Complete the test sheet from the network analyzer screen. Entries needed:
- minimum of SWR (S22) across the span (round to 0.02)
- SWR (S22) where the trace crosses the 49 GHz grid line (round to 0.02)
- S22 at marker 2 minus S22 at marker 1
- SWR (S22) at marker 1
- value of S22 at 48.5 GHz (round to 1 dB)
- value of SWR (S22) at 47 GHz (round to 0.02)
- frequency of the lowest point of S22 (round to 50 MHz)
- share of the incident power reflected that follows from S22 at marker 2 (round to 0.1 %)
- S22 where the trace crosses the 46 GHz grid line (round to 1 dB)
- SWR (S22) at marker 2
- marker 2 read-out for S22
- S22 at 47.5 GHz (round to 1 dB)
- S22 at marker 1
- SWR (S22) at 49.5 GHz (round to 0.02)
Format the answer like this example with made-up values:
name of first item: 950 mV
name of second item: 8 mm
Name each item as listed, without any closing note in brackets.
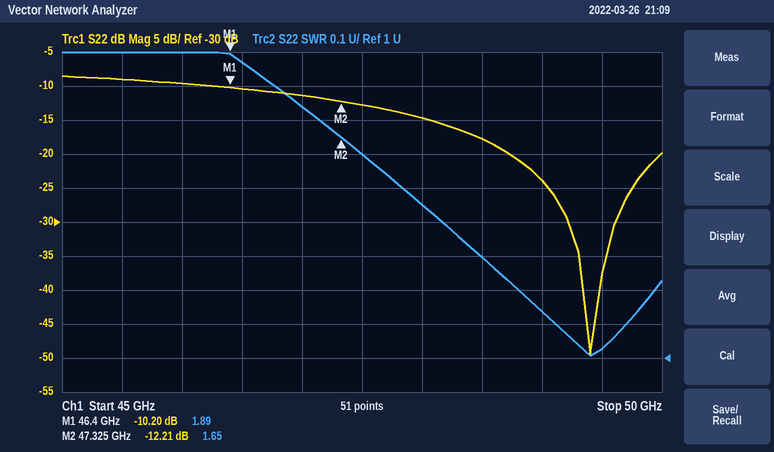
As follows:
minimum of SWR (S22) across the span: 1.00
SWR (S22) where the trace crosses the 49 GHz grid line: 1.14
S22 at marker 2 minus S22 at marker 1: -2.01 dB
SWR (S22) at marker 1: 1.89
value of S22 at 48.5 GHz: -18 dB
value of SWR (S22) at 47 GHz: 1.74
frequency of the lowest point of S22: 49.40 GHz
share of the incident power reflected that follows from S22 at marker 2: 6.0 %
S22 where the trace crosses the 46 GHz grid line: -10 dB
SWR (S22) at marker 2: 1.65
marker 2 read-out for S22: -12.21 dB
S22 at 47.5 GHz: -13 dB
S22 at marker 1: -10.20 dB
SWR (S22) at 49.5 GHz: 1.02
